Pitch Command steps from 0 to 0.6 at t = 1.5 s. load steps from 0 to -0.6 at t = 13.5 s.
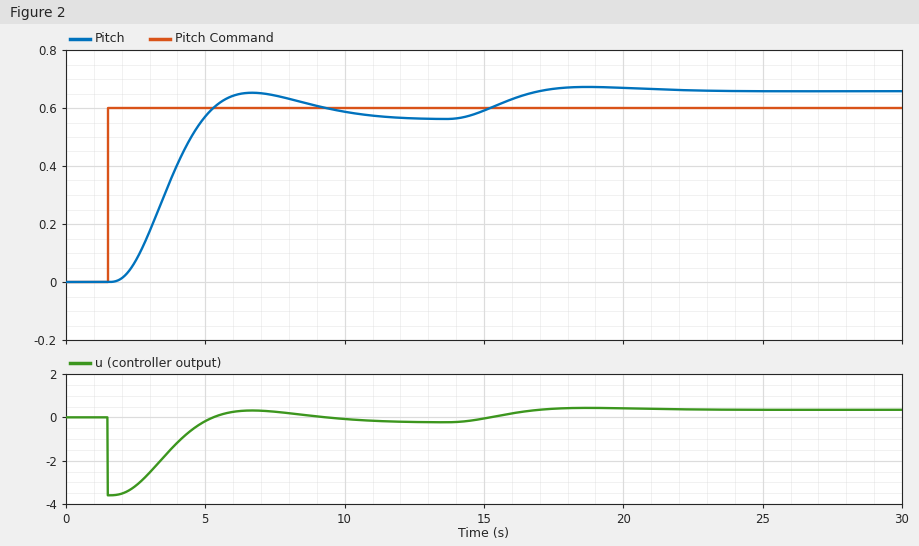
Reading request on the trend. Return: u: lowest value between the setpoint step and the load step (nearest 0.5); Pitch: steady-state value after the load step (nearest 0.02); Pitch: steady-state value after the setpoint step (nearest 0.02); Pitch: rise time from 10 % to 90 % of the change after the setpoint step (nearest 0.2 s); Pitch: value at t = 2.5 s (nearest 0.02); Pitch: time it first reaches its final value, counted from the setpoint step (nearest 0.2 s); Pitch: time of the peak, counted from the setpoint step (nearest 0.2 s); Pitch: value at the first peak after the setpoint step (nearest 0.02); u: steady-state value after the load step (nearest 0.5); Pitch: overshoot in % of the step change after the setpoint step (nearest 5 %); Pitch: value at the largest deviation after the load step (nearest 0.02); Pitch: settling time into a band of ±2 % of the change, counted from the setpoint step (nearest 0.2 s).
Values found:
-3.5
0.66
0.56
2.2 s
0.08
3.4 s
5.2 s
0.66
0.5
15 %
0.68
9.4 s
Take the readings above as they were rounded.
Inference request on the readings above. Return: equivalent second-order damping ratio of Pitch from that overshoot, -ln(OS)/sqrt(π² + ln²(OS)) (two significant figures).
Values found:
0.52
